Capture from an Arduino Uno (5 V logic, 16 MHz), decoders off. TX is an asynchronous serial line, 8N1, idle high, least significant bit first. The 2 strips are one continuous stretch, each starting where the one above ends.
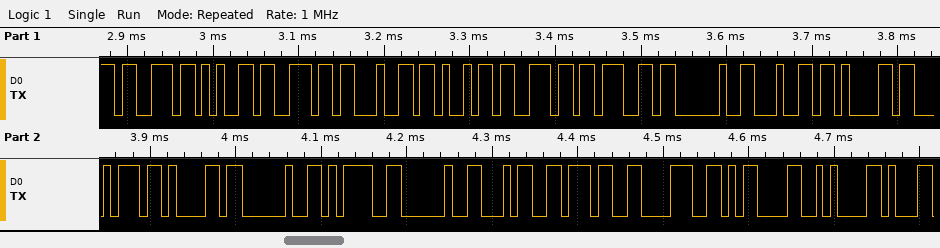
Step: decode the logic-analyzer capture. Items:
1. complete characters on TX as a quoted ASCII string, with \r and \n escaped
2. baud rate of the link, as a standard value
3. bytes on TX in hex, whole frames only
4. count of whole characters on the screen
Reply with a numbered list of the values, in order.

1. "sending data = 478\r\n"
2. 115200 baud
3. 73 65 6E 64 69 6E 67 20 64 61 74 61 20 3D 20 34 37 38 0D 0A
4. 20
